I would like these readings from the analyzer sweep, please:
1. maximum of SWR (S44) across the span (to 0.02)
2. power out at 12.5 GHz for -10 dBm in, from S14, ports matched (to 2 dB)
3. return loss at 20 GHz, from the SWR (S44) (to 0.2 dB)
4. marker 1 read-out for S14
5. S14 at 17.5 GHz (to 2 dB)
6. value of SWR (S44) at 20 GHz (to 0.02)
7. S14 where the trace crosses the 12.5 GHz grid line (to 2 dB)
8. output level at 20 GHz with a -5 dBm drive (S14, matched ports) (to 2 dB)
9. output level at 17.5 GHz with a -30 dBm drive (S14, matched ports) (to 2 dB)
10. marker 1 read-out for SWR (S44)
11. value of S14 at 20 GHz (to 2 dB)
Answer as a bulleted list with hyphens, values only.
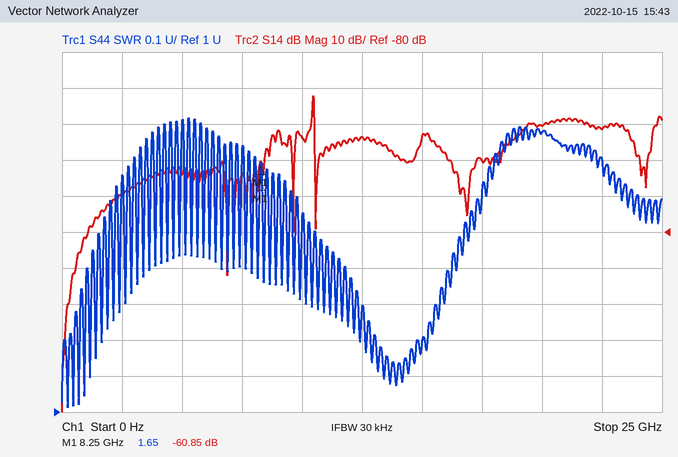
- 1.82
- -64 dBm
- 11.0 dB
- -60.85 dB
- -60 dB
- 1.78
- -54 dB
- -56 dBm
- -90 dBm
- 1.65
- -50 dB
